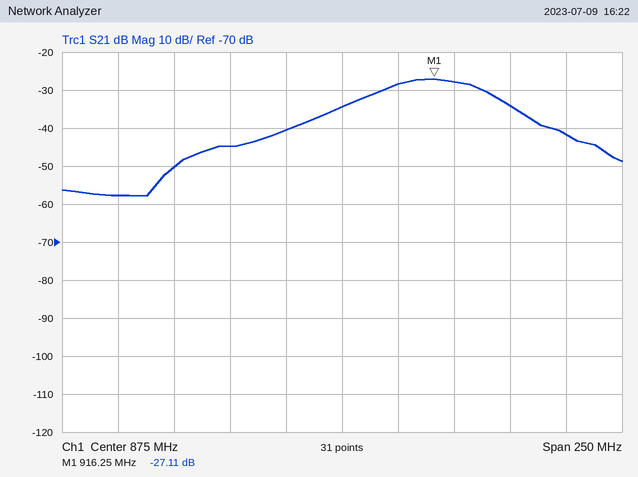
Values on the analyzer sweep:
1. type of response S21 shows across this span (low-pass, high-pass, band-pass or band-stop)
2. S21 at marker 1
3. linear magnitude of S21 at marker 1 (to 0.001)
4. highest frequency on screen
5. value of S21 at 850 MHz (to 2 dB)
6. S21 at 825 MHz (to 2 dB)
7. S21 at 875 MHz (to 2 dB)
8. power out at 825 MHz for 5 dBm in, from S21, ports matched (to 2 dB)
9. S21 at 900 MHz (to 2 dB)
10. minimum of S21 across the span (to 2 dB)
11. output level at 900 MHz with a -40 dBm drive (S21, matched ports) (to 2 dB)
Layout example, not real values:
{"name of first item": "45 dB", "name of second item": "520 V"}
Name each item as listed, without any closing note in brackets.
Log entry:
{"type of response S21 shows across this span": "band-pass", "S21 at marker 1": "-27.11 dB", "linear magnitude of S21 at marker 1": "0.044", "highest frequency on screen": "1 GHz", "value of S21 at 850 MHz": "-40 dB", "S21 at 825 MHz": "-44 dB", "S21 at 875 MHz": "-34 dB", "power out at 825 MHz for 5 dBm in, from S21, ports matched": "-40 dBm", "S21 at 900 MHz": "-28 dB", "minimum of S21 across the span": "-58 dB", "output level at 900 MHz with a -40 dBm drive (S21, matched ports)": "-68 dBm"}
